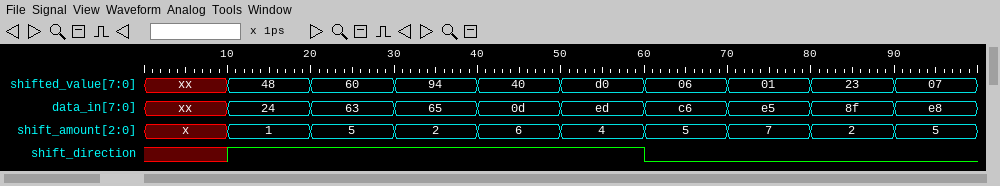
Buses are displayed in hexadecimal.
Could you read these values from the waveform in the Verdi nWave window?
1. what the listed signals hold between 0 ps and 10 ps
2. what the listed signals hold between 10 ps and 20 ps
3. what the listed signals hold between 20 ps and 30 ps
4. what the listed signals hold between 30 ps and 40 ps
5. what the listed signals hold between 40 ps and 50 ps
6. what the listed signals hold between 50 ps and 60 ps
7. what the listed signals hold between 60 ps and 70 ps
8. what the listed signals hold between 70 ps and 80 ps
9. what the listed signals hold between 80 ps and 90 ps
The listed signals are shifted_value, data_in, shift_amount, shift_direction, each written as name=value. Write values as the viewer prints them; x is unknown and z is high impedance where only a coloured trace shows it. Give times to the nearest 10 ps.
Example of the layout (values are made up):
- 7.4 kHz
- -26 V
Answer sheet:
- shifted_value=xx, data_in=xx, shift_amount=x, shift_direction=x
- shifted_value=48, data_in=24, shift_amount=1, shift_direction=1
- shifted_value=60, data_in=63, shift_amount=5, shift_direction=1
- shifted_value=94, data_in=65, shift_amount=2, shift_direction=1
- shifted_value=40, data_in=0d, shift_amount=6, shift_direction=1
- shifted_value=d0, data_in=ed, shift_amount=4, shift_direction=1
- shifted_value=06, data_in=c6, shift_amount=5, shift_direction=0
- shifted_value=01, data_in=e5, shift_amount=7, shift_direction=0
- shifted_value=23, data_in=8f, shift_amount=2, shift_direction=0
